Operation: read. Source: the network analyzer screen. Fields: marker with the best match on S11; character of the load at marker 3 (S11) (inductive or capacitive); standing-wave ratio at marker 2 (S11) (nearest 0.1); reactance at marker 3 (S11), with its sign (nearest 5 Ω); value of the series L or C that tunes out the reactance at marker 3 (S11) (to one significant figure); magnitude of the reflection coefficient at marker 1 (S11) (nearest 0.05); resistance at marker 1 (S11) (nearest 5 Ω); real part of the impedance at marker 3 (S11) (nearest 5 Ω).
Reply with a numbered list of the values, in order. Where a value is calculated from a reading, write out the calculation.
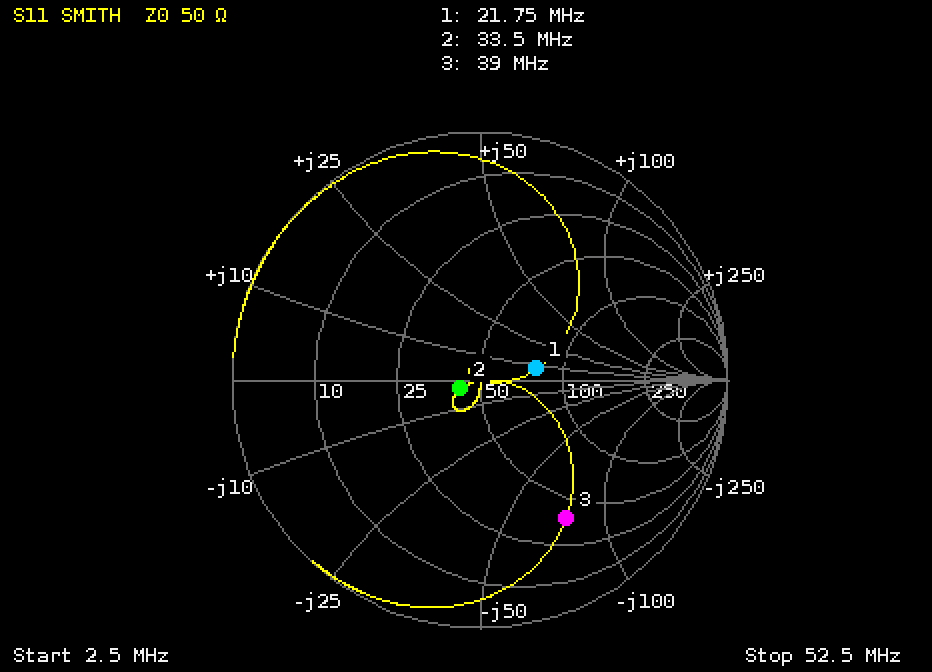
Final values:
1. marker 2
2. capacitive
3. 1.2
4. -75 Ω
5. L = 75 Ω/(2π × 39 MHz) ≈ 306 nH, so 300 nH to one significant figure
6. 0.25
7. 80 Ω
8. 40 Ω
